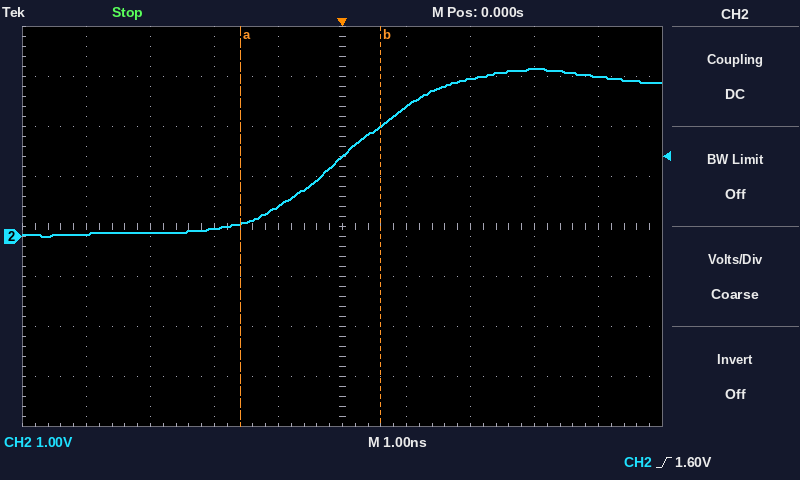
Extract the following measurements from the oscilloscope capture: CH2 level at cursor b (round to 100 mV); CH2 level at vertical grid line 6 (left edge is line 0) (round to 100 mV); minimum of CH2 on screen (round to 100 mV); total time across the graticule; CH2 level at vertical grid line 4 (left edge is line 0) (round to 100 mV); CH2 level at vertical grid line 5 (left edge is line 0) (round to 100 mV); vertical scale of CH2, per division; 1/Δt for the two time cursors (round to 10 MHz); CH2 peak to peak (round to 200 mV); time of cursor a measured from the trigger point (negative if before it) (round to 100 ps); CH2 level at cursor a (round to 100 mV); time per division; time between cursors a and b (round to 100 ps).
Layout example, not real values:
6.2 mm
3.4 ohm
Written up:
2.2 V
2.6 V
0.0 V
10 ns
600 mV
1.6 V
1 V
450 MHz
3.4 V
-1.6 ns
300 mV
1 ns
2.2 ns
